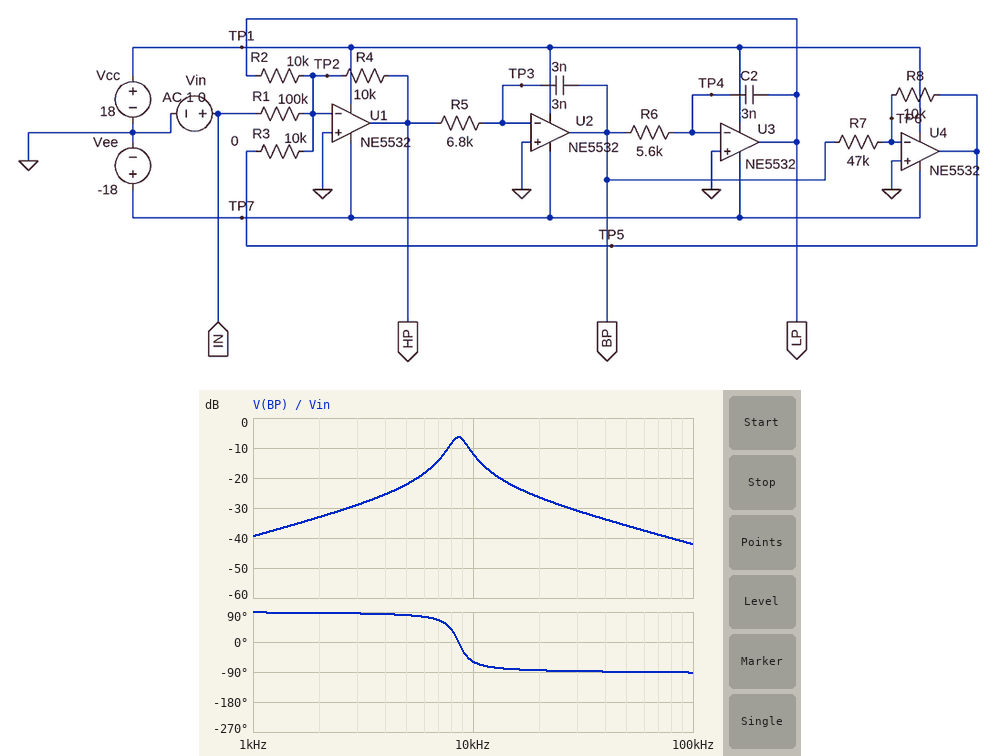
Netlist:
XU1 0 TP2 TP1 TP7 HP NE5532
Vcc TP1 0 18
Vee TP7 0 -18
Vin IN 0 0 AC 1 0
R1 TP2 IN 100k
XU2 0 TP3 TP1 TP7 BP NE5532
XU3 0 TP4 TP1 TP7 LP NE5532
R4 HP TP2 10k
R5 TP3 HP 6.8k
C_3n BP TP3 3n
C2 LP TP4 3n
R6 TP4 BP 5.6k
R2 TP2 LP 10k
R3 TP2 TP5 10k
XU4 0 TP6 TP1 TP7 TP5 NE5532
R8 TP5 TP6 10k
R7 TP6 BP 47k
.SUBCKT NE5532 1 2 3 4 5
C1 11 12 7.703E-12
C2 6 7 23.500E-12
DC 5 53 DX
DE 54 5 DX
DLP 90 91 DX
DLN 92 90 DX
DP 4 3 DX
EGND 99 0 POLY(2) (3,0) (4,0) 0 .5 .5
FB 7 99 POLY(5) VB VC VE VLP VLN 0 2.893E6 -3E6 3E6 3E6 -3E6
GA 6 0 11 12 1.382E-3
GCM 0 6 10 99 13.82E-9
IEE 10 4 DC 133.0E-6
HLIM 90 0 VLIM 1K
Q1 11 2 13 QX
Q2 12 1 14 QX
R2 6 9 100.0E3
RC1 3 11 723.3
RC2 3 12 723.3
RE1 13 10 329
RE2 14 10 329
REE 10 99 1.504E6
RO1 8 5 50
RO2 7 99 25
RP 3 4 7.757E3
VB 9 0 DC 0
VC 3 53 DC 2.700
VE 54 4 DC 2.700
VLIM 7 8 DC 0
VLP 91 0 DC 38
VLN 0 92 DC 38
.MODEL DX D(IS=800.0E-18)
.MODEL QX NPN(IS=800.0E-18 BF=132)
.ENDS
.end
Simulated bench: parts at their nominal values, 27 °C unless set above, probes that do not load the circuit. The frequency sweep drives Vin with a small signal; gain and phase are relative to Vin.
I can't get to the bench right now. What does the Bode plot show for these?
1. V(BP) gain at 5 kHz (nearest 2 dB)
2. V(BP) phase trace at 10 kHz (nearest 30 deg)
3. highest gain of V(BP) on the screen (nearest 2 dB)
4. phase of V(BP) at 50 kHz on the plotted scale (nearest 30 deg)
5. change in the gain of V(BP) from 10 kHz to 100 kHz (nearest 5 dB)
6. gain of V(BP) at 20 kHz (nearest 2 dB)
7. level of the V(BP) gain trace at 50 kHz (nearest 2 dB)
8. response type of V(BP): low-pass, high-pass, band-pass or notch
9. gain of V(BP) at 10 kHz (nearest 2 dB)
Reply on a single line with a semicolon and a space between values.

-22 dB; -60 deg; -6 dB; -90 deg; -30 dB; -26 dB; -36 dB; band-pass; -12 dB
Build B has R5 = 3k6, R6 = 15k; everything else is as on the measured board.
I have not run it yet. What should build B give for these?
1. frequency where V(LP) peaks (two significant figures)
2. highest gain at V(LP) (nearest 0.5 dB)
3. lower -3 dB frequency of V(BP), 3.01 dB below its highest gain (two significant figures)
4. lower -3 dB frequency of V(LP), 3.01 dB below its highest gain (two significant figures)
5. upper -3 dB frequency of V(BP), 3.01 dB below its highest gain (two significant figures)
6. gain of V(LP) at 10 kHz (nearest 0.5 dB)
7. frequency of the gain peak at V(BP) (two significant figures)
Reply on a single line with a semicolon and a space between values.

6.9 kHz; -12.5 dB; 5.8 kHz; 5.0 kHz; 8.9 kHz; -21.0 dB; 7.2 kHz
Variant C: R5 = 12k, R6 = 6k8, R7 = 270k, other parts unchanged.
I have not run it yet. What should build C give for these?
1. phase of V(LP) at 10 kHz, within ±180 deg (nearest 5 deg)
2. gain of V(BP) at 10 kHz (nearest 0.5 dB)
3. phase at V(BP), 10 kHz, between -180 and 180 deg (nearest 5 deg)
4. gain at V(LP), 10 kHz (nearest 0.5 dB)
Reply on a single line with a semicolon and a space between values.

0 deg; -23.5 dB; -90 deg; -25.5 dB
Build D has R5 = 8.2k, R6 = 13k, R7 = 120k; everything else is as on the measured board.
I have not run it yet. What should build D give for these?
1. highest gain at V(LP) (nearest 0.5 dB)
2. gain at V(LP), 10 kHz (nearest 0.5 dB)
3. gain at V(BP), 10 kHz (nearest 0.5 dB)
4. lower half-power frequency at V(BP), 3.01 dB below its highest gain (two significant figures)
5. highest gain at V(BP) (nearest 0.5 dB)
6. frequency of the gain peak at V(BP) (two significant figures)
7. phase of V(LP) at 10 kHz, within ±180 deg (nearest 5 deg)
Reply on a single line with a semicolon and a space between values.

0 dB; -29.0 dB; -21.0 dB; 4.9 kHz; 2.0 dB; 5.1 kHz; 5 deg
